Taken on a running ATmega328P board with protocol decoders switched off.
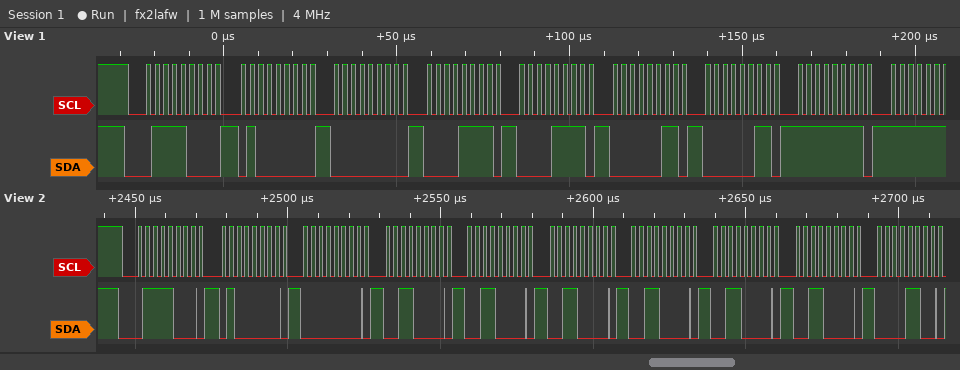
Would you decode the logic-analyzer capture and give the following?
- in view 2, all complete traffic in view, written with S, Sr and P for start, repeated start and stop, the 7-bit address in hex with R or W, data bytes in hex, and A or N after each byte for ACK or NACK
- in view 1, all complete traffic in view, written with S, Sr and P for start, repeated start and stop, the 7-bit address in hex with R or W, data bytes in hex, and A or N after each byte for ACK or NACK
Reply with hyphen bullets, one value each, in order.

- S 3CW A 40 A 00 A 30 A 30 A 30 A 30 A 30 A 30 A 0C A
- S 3CW A 40 A 00 A 0F A 0F A 03 A 03 A FF A
